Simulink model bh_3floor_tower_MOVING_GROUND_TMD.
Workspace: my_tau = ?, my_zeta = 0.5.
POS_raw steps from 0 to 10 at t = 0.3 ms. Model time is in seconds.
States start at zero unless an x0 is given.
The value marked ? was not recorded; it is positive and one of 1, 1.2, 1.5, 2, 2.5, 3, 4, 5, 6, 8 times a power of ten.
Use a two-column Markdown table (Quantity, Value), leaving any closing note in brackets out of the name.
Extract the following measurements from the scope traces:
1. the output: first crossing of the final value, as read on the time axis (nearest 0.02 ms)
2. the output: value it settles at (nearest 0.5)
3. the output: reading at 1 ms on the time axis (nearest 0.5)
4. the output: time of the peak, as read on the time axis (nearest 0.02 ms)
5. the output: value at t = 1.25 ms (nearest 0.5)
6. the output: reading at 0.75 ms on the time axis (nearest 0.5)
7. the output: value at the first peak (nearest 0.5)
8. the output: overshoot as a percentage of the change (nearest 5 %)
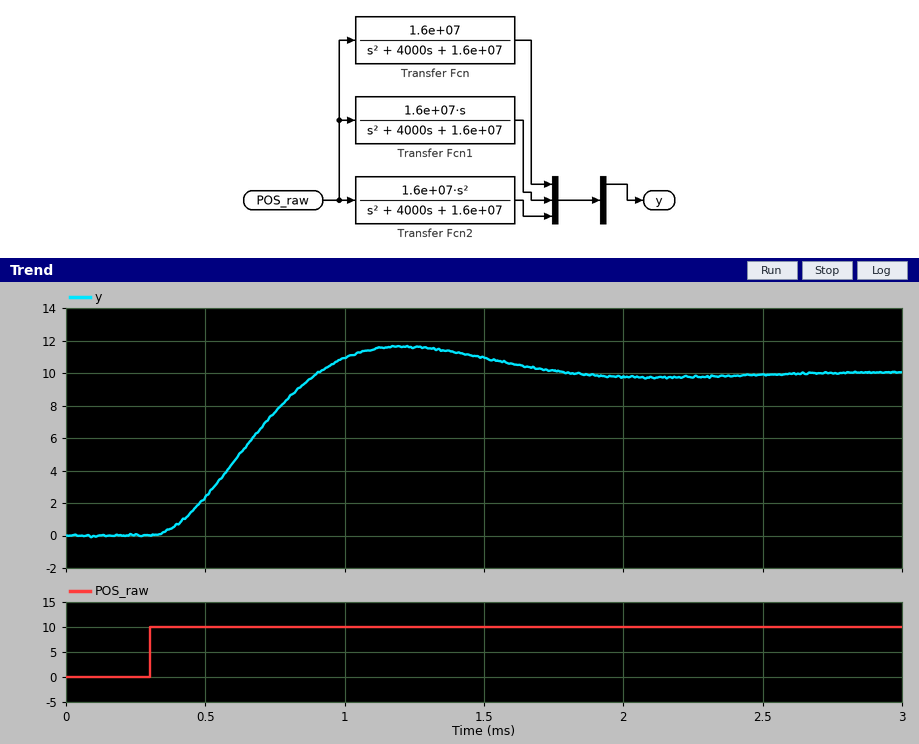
| Quantity | Value |
|---|---|
| the output: first crossing of the final value, as read on the time axis | 0.90 ms |
| the output: value it settles at | 10.0 |
| the output: reading at 1 ms on the time axis | 11.0 |
| the output: time of the peak, as read on the time axis | 1.20 ms |
| the output: value at t = 1.25 ms | 11.5 |
| the output: reading at 0.75 ms on the time axis | 7.5 |
| the output: value at the first peak | 11.5 |
| the output: overshoot as a percentage of the change | 15 % |
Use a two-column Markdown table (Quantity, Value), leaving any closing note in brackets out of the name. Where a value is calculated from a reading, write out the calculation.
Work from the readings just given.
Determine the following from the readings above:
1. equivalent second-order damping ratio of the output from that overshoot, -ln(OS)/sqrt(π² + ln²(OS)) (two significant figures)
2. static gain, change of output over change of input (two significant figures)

| Quantity | Value |
|---|---|
| equivalent second-order damping ratio of the output from that overshoot, -ln(OS)/sqrt(π² + ln²(OS)) | ln(0.15) = -1.897; 1.897 / sqrt(9.870 + 3.599) = 0.52 |
| static gain, change of output over change of input | (10 - 0) / (10 - 0) = 1.0 |
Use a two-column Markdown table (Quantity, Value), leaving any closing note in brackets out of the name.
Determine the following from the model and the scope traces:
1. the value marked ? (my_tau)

| Quantity | Value |
|---|---|
| the value marked ? | 0.0005 |
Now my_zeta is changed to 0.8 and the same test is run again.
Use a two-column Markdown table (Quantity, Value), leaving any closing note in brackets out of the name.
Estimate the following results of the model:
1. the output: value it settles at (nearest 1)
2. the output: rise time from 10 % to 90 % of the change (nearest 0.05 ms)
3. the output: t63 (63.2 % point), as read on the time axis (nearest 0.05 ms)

| Quantity | Value |
|---|---|
| the output: value it settles at | 10 |
| the output: rise time from 10 % to 90 % of the change | 1.00 ms |
| the output: t63 (63.2 % point), as read on the time axis | 1.05 ms |
